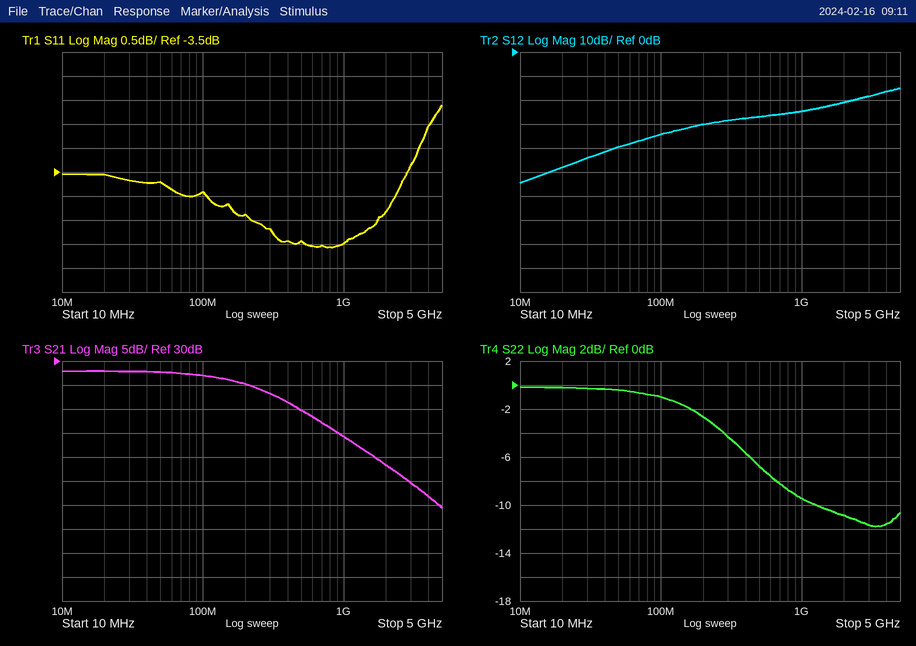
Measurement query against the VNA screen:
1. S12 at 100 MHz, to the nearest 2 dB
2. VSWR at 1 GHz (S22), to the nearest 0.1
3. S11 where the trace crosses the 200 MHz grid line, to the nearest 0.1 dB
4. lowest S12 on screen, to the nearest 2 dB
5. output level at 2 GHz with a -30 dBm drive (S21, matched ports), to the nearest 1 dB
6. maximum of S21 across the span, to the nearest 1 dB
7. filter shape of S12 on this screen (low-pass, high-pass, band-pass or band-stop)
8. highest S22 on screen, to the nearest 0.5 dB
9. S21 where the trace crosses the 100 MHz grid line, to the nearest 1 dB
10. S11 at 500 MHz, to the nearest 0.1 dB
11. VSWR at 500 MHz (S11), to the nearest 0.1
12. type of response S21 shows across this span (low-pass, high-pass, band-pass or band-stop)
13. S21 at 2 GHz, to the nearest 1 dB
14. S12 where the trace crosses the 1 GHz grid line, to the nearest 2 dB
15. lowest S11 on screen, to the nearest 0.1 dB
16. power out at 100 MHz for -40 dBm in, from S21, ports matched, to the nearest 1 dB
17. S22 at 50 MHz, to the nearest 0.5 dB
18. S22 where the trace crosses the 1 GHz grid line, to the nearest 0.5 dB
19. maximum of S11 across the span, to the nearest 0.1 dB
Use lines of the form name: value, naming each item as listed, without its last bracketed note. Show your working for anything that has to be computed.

S12 at 100 MHz, to the nearest 2 dB: -34 dB
VSWR at 1 GHz (S22), to the nearest 0.1: |Γ| = 10^(-9.5/20) = 0.3350; VSWR = (1 + 0.3350)/(1 − 0.3350) ≈ 2.0
S11 where the trace crosses the 200 MHz grid line, to the nearest 0.1 dB: -4.4 dB
lowest S12 on screen, to the nearest 2 dB: -54 dB
output level at 2 GHz with a -30 dBm drive (S21, matched ports), to the nearest 1 dB: -30 dBm + (8 dB) = -22 dBm
maximum of S21 across the span, to the nearest 1 dB: 28 dB
filter shape of S12 on this screen: high-pass
highest S22 on screen, to the nearest 0.5 dB: 0.0 dB
S21 where the trace crosses the 100 MHz grid line, to the nearest 1 dB: 27 dB
S11 at 500 MHz, to the nearest 0.1 dB: -4.9 dB
VSWR at 500 MHz (S11), to the nearest 0.1: |Γ| = 10^(-4.9/20) = 0.5689; VSWR = (1 + 0.5689)/(1 − 0.5689) ≈ 3.6
type of response S21 shows across this span: low-pass
S21 at 2 GHz, to the nearest 1 dB: 8 dB
S12 where the trace crosses the 1 GHz grid line, to the nearest 2 dB: -24 dB
lowest S11 on screen, to the nearest 0.1 dB: -5.1 dB
power out at 100 MHz for -40 dBm in, from S21, ports matched, to the nearest 1 dB: -40 dBm + (27 dB) = -13 dBm
S22 at 50 MHz, to the nearest 0.5 dB: -0.5 dB
S22 where the trace crosses the 1 GHz grid line, to the nearest 0.5 dB: -9.5 dB
maximum of S11 across the span, to the nearest 0.1 dB: -2.1 dB
